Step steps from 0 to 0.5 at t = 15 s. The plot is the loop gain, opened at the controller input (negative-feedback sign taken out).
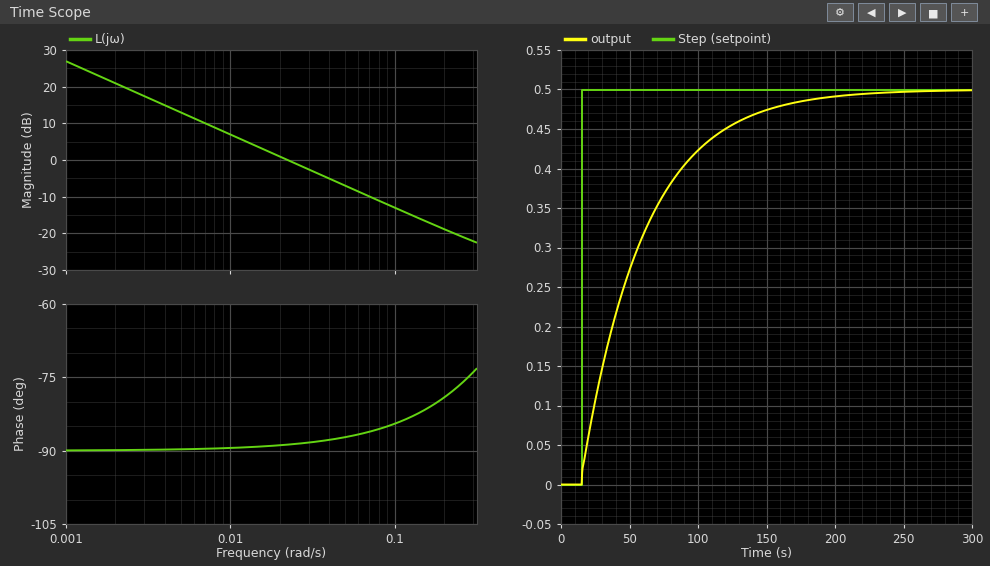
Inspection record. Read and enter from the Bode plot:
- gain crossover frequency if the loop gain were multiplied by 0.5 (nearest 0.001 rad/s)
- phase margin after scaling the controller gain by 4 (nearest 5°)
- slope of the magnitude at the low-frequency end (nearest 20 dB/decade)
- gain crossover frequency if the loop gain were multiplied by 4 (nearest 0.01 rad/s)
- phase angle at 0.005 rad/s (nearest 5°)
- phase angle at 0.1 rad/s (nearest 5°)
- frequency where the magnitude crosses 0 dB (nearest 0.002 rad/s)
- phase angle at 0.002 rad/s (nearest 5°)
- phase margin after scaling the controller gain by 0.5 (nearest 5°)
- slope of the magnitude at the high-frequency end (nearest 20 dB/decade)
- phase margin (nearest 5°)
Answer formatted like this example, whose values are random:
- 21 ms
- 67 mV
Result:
- 0.011 rad/s
- 95°
- -20 dB/decade
- 0.09 rad/s
- -90°
- -85°
- 0.022 rad/s
- -90°
- 90°
- -20 dB/decade
- 90°
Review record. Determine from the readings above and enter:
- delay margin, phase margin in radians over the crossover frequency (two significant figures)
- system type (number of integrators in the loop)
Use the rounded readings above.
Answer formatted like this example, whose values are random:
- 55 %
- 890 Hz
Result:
- 71 s
- 1
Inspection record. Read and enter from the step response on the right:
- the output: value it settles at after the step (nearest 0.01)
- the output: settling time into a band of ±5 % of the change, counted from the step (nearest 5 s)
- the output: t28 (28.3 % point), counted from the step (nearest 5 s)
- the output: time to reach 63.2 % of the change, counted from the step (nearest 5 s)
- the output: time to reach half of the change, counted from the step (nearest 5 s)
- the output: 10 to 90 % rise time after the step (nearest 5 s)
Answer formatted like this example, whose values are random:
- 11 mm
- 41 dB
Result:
- 0.50
- 135 s
- 15 s
- 45 s
- 30 s
- 100 s
